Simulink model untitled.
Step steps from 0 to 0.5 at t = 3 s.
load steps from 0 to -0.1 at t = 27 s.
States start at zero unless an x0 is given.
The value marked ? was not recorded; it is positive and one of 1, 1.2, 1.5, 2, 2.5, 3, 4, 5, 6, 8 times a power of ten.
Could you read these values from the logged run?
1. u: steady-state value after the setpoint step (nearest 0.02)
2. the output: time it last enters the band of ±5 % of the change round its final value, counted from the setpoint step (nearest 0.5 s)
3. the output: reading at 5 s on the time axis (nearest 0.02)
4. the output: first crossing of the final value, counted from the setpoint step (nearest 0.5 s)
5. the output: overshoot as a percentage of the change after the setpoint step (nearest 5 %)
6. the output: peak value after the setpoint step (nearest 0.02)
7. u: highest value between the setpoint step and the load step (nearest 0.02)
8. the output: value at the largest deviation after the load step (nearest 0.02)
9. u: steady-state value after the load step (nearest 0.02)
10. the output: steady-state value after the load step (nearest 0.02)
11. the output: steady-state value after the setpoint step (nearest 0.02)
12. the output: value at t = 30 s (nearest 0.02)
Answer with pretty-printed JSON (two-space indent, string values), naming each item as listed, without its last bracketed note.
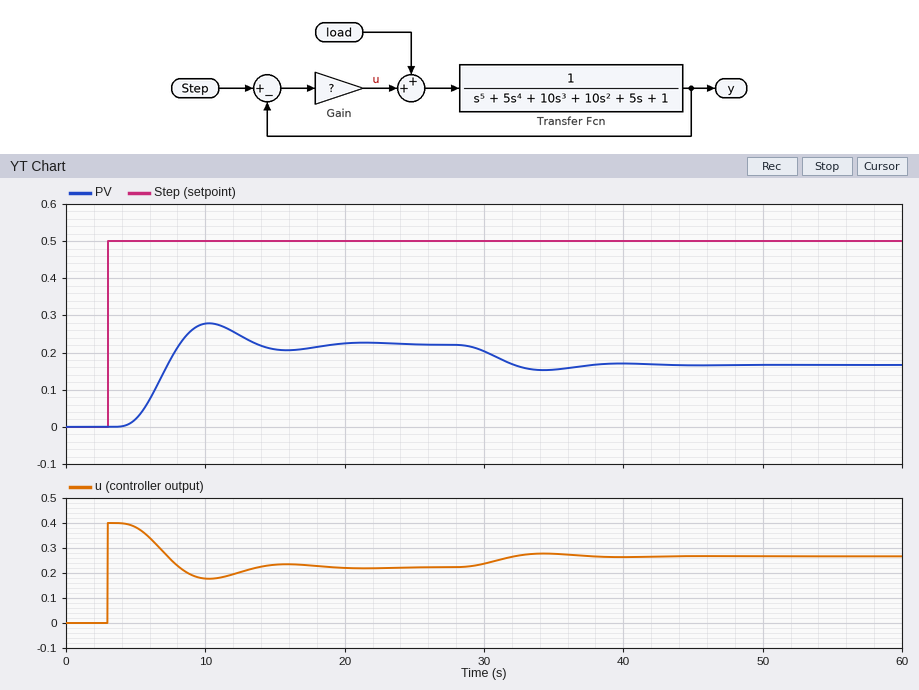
{
  "u: steady-state value after the setpoint step": "0.22",
  "the output: time it last enters the band of ±5 % of the change round its final value, counted from the setpoint step": "14.5 s",
  "the output: reading at 5 s on the time axis": "0.02",
  "the output: first crossing of the final value, counted from the setpoint step": "5.0 s",
  "the output: overshoot as a percentage of the change after the setpoint step": "25 %",
  "the output: peak value after the setpoint step": "0.28",
  "u: highest value between the setpoint step and the load step": "0.40",
  "the output: value at the largest deviation after the load step": "0.16",
  "u: steady-state value after the load step": "0.26",
  "the output: steady-state value after the load step": "0.16",
  "the output: steady-state value after the setpoint step": "0.22",
  "the output: value at t = 30 s": "0.20"
}
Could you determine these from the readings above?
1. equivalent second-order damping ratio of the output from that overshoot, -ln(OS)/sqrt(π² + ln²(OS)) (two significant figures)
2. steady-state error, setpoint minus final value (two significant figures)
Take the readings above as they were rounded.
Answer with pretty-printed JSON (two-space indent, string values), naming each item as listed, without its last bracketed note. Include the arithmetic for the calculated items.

{
  "equivalent second-order damping ratio of the output from that overshoot, -ln(OS)/sqrt(π² + ln²(OS))": "ln(0.25) = -1.386; 1.386 / sqrt(9.870 + 1.922) = 0.40",
  "steady-state error, setpoint minus final value": "0.5 - 0.22 = 0.28"
}
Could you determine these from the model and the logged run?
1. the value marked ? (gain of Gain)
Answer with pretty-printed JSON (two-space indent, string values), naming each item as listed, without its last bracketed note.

{
  "the value marked ?": "0.8"
}
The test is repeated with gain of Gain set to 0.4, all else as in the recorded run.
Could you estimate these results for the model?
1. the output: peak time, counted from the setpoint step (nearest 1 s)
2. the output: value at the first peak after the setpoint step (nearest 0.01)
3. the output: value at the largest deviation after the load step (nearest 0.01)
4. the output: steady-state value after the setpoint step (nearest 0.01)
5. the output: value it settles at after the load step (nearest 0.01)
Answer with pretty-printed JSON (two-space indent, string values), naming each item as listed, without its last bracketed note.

{
  "the output: peak time, counted from the setpoint step": "8 s",
  "the output: value at the first peak after the setpoint step": "0.16",
  "the output: value at the largest deviation after the load step": "0.06",
  "the output: steady-state value after the setpoint step": "0.14",
  "the output: value it settles at after the load step": "0.07"
}
